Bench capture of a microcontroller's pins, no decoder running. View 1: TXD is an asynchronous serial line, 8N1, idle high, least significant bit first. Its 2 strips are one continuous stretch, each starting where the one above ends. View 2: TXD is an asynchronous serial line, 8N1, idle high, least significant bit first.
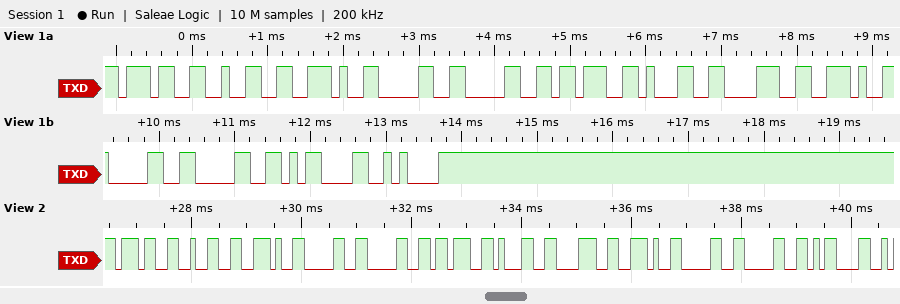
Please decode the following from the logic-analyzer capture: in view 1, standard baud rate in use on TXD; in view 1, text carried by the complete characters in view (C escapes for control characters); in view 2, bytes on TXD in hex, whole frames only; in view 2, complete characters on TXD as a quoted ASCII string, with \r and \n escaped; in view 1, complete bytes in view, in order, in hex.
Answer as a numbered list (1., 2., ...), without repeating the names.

1. 9600 baud
2. "72.00;18.00\r\n"
3. 37 32 2E 30 30 3B 31 38 2E 30 30 0D
4. "72.00;18.00\r"
5. 0x37 0x32 0x2E 0x30 0x30 0x3B 0x31 0x38 0x2E 0x30 0x30 0x0D 0x0A
